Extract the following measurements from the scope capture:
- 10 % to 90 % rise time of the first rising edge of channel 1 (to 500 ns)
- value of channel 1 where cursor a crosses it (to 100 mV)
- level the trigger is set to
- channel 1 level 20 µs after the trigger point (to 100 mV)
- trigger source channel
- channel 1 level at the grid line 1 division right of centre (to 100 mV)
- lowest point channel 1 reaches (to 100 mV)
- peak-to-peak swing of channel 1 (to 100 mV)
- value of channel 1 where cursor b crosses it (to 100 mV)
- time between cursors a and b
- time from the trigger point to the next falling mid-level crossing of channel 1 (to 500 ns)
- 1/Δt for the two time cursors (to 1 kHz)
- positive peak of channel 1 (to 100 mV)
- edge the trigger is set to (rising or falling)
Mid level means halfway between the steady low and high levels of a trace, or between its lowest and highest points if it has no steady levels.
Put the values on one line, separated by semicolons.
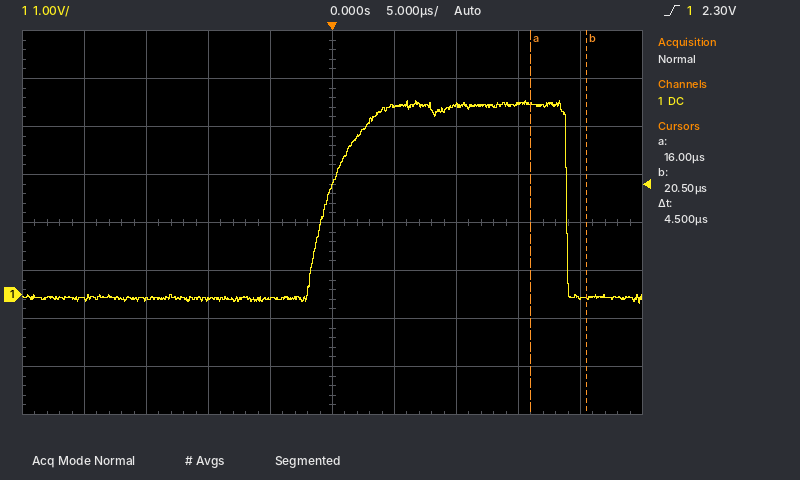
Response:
4.5 µs; 4.0 V; 2.30 V; -100 mV; channel 1; 3.9 V; -200 mV; 4.2 V; -100 mV; 4.5 µs; 19.0 µs; 222 kHz; 4.0 V; rising
